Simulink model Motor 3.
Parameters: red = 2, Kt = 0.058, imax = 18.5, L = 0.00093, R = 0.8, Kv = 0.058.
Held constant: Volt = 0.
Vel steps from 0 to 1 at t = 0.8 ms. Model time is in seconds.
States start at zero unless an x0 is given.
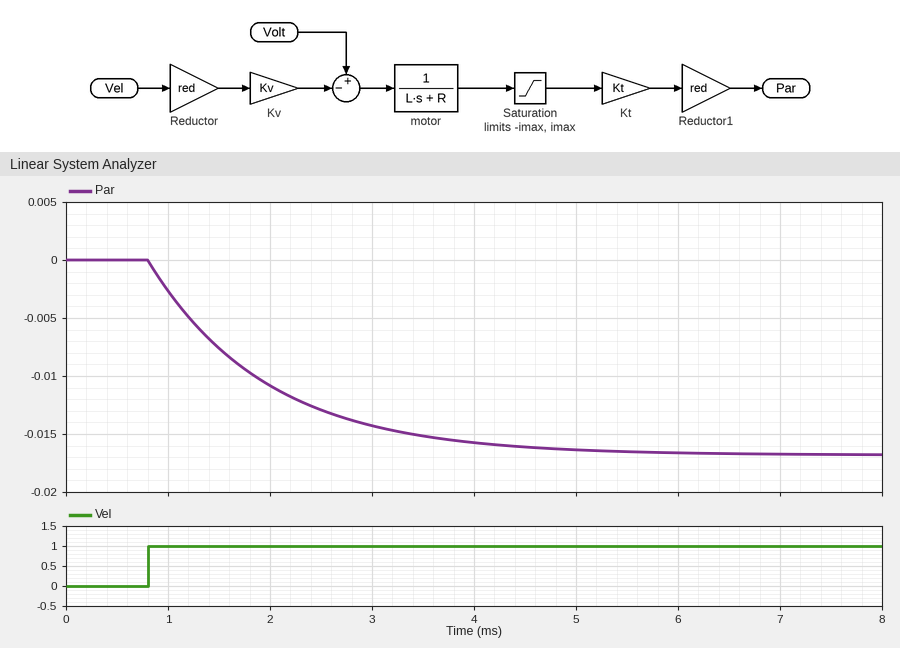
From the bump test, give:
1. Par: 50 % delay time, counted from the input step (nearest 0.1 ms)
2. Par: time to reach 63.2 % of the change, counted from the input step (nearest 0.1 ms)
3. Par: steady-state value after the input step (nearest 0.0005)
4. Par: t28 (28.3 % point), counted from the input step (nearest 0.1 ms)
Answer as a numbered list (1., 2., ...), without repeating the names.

1. 0.8 ms
2. 1.2 ms
3. -0.0170
4. 0.4 ms
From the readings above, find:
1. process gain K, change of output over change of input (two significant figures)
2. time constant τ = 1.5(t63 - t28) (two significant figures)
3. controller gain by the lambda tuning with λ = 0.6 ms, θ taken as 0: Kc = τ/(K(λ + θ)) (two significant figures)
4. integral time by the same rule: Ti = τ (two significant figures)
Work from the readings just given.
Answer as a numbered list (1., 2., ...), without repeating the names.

1. -0.017
2. 1.2 ms
3. -120
4. 1.2 ms
